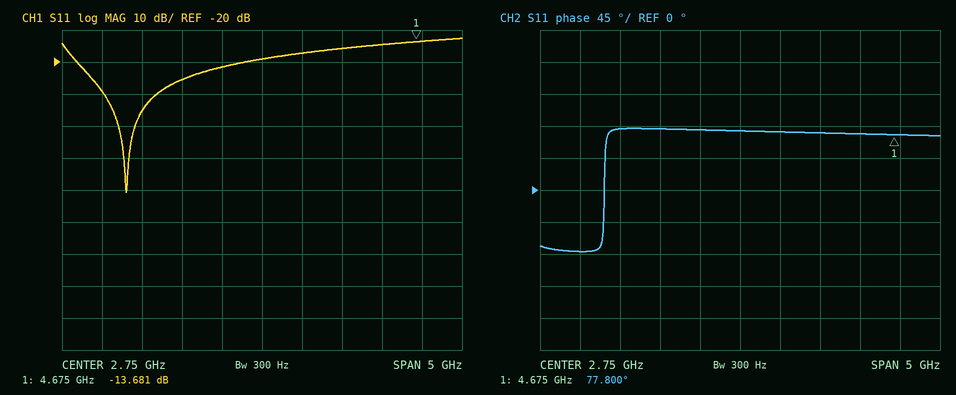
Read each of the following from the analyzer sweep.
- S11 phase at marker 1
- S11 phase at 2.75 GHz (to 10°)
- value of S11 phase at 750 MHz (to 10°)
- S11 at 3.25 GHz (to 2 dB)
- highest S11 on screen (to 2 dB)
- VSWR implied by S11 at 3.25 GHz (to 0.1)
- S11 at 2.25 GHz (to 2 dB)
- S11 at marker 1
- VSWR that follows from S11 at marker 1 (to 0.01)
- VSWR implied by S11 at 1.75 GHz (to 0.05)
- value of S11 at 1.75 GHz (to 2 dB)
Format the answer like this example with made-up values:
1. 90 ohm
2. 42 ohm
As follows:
1. 77.800°
2. 80°
3. -90°
4. -18 dB
5. -12 dB
6. 1.3
7. -22 dB
8. -13.681 dB
9. 1.52
10. 1.10
11. -26 dB
